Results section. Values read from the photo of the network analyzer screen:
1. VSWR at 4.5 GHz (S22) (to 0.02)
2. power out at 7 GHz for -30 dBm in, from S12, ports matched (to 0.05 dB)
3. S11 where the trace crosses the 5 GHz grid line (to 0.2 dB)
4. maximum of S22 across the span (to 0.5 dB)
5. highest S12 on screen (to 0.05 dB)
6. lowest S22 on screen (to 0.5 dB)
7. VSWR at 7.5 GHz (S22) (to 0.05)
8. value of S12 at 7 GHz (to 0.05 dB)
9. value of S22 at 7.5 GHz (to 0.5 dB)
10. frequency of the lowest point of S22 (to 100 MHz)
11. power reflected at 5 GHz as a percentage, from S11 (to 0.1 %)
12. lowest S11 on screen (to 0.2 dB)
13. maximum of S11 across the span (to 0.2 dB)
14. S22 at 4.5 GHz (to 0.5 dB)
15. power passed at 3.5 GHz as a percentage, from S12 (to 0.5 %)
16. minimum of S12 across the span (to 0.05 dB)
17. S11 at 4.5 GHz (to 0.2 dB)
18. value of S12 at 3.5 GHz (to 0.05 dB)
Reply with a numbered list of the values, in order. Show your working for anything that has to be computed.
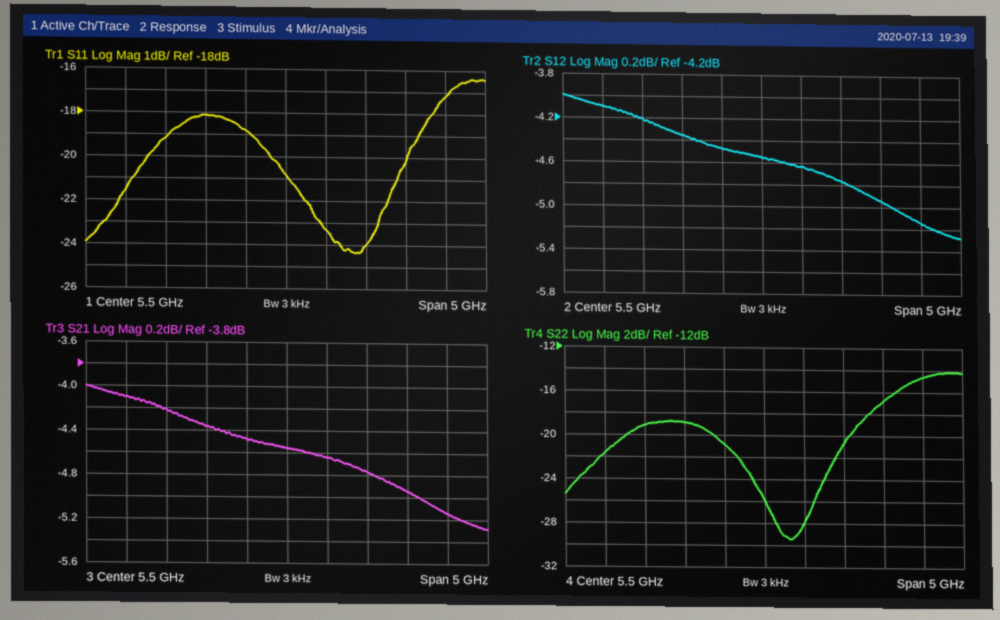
1. |Γ| = 10^(-19/20) = 0.1122; VSWR = (1 + 0.1122)/(1 − 0.1122) ≈ 1.25, so 1.26 to the nearest 0.02
2. -30 dBm + (-4.95 dB) = -34.95 dBm
3. -18.8 dB
4. -14.0 dB
5. -4.00 dB
6. -29.5 dB
7. |Γ| = 10^(-14.5/20) = 0.1884; VSWR = (1 + 0.1884)/(1 − 0.1884) ≈ 1.46, so 1.45 to the nearest 0.05
8. -4.95 dB
9. -14.5 dB
10. 5.8 GHz
11. 10^(-18.8/10) ≈ 1.3 %
12. -24.4 dB
13. -16.4 dB
14. -19.0 dB
15. 10^(-4.1/10) ≈ 38.9 %, so 39.0 % to the nearest 0.5 %
16. -5.30 dB
17. -18.2 dB
18. -4.10 dB
